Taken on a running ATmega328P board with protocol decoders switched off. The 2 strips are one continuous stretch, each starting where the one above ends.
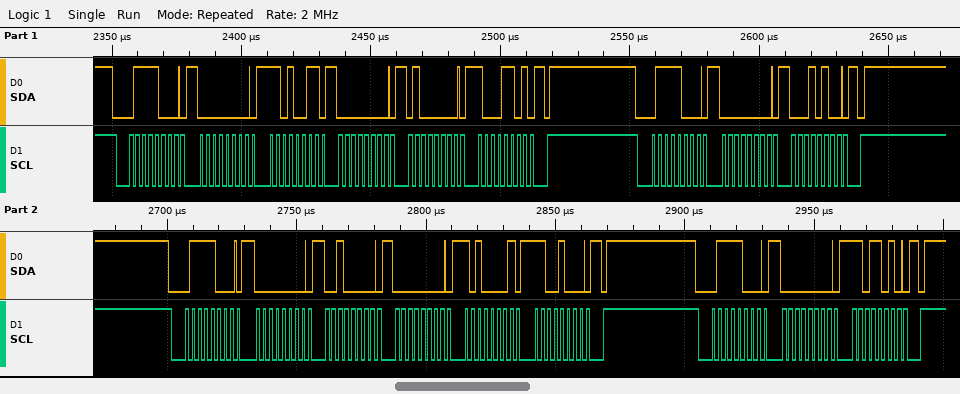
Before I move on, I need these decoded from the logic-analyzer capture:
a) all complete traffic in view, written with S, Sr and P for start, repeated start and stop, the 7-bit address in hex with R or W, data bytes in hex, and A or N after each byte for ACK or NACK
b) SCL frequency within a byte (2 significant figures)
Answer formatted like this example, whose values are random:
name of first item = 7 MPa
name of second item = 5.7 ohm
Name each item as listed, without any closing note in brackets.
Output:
all complete traffic in view, written with S, Sr and P for start, repeated start and stop, the 7-bit address in hex with R or W, data bytes in hex, and A or N after each byte for ACK or NACK = S 3CW A 00 A D3 A 00 A 40 A 8D A P S 3CW A 00 A 14 A P S 3CW A 00 A 20 A 00 A A1 A C8 A P S 3CW A 00 A DA A P
SCL frequency within a byte = 400 kHz
